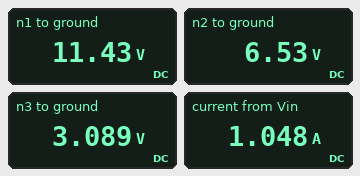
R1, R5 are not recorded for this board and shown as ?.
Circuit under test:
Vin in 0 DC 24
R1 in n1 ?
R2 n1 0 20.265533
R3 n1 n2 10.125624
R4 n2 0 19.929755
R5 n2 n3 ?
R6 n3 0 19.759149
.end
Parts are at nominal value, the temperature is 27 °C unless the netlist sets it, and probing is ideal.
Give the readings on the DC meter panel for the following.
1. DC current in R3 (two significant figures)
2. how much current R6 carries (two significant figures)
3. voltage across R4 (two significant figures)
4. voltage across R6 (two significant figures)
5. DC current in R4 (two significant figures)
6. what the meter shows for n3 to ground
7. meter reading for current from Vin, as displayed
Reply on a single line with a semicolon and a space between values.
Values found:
480 mA; 160 mA; 6.5 V; 3.1 V; 330 mA; 3.089 V; 1.048 A
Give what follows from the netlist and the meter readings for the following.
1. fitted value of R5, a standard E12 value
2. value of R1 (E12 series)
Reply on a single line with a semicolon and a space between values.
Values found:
22 Ω; 12 Ω
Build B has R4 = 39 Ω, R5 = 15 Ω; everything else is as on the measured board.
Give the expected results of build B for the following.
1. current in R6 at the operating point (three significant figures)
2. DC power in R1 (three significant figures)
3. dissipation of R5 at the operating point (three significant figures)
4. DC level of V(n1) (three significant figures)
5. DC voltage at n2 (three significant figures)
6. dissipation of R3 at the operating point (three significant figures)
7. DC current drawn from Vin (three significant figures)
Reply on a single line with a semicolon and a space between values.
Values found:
221 mA; 12.2 W; 734 mW; 11.9 V; 7.69 V; 1.77 W; 1.01 A
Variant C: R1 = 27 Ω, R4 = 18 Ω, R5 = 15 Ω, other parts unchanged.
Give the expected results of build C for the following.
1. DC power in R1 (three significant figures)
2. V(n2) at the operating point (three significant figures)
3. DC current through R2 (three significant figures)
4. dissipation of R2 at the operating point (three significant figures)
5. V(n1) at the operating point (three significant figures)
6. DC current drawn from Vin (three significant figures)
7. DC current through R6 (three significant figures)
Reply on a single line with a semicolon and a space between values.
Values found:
11.0 W; 3.64 V; 333 mA; 2.24 W; 6.74 V; 639 mA; 105 mA
